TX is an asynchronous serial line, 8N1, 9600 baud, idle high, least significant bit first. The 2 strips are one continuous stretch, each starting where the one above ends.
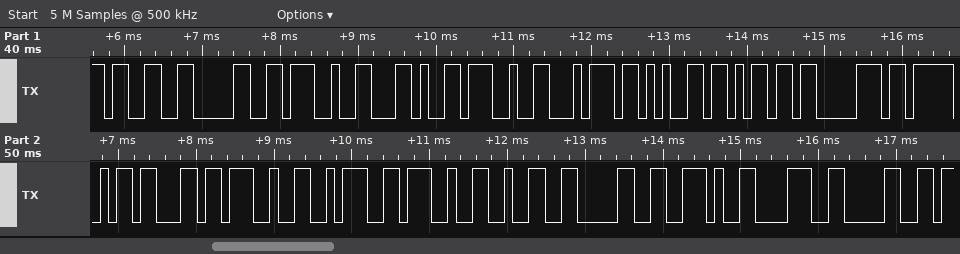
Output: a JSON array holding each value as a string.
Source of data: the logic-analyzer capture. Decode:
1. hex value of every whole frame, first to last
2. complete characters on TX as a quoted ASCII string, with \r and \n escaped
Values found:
["33 30 27 2C 27 74 65 6D 70 5F 63 27 3A 27 32 30 2E 38 30", "\"30','temp_c':'20.80\""]
